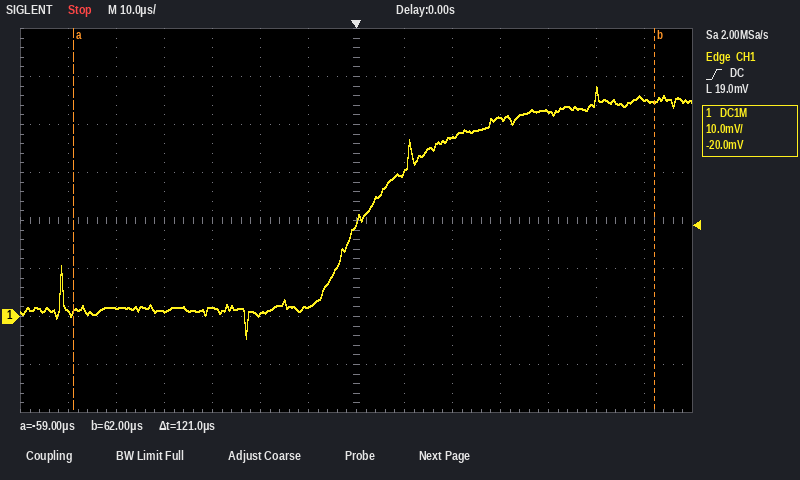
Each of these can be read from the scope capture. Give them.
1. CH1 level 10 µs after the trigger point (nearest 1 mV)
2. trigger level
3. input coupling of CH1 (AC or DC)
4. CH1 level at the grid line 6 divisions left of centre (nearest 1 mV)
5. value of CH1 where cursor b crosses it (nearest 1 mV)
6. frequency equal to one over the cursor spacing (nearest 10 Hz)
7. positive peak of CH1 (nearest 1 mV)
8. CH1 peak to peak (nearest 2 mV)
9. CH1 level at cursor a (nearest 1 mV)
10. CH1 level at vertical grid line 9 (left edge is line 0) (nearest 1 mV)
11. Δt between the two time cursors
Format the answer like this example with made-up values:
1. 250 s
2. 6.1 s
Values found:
1. 30 mV
2. 19.0 mV
3. DC
4. 1 mV
5. 45 mV
6. 8.26 kHz
7. 48 mV
8. 52 mV
9. 1 mV
10. 37 mV
11. 121 µs
